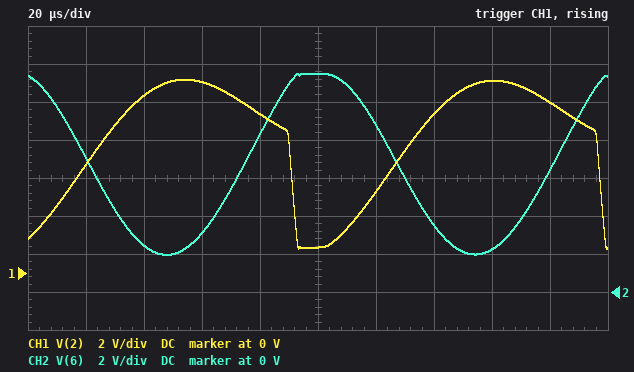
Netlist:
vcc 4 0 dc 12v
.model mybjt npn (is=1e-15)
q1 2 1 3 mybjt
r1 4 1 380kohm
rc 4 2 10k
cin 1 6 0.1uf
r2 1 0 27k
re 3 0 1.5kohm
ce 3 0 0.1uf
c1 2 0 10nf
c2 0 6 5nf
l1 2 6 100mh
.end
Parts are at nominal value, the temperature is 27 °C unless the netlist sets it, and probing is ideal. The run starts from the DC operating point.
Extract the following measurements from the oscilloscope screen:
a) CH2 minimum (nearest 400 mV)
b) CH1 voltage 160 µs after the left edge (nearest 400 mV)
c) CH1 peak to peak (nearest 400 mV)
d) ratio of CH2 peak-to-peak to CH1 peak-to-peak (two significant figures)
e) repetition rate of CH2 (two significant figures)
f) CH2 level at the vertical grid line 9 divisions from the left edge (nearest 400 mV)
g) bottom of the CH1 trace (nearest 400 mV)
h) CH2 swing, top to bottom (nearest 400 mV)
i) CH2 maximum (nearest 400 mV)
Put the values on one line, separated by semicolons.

2.0 V; 10.0 V; 8.8 V; 1.1; 9.4 kHz; 6.4 V; 1.2 V; 9.6 V; 11.6 V
